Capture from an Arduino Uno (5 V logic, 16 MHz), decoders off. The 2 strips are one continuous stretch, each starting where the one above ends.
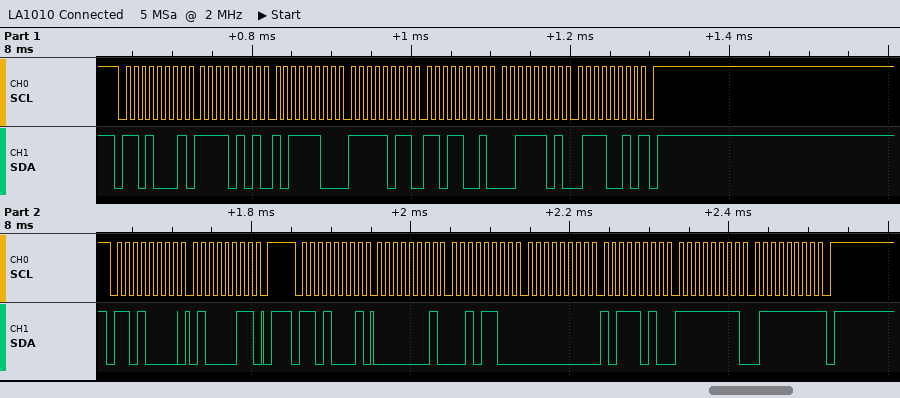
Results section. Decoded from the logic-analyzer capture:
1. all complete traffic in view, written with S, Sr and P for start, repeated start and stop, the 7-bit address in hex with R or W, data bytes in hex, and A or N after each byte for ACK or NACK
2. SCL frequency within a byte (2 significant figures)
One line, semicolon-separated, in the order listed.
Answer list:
S 68R A F5 A BC A FB A D9 A 3D A 72 N P S 68W A 43 A P S 68R A 01 A 2C A 00 A BA A FF A 7F N P; 100 kHz
